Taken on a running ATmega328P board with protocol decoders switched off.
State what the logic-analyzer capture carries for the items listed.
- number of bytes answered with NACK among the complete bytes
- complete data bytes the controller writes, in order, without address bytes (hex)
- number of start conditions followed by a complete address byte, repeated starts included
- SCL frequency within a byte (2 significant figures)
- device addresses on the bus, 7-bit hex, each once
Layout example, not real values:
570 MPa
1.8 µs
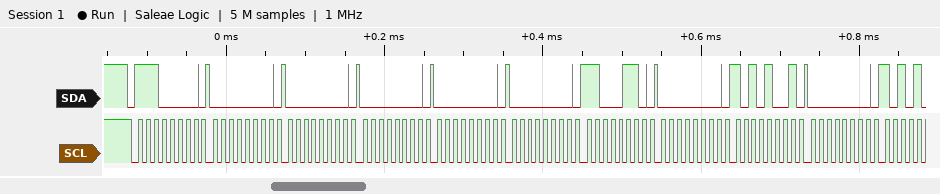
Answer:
0
00 00 00 00 00 C6 00 A9 00
1
100 kHz
0x70
